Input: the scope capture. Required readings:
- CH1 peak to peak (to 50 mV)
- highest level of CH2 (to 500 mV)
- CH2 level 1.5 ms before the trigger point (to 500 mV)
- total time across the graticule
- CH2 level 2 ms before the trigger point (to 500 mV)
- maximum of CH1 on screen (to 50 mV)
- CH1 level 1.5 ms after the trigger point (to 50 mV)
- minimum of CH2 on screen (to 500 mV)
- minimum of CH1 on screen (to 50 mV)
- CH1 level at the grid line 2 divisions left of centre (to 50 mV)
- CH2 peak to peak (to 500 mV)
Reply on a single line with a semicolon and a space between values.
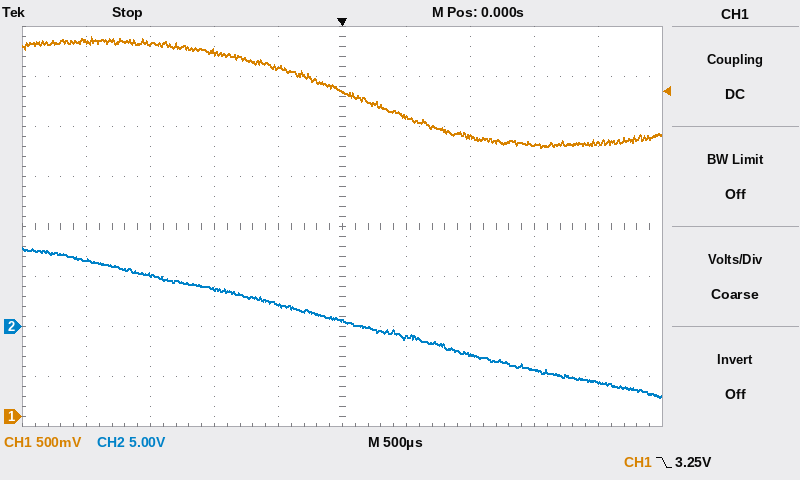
1.10 V; 8.0 V; 5.0 V; 5 ms; 6.5 V; 3.80 V; 2.70 V; -7.0 V; 2.70 V; 3.65 V; 15.0 V
